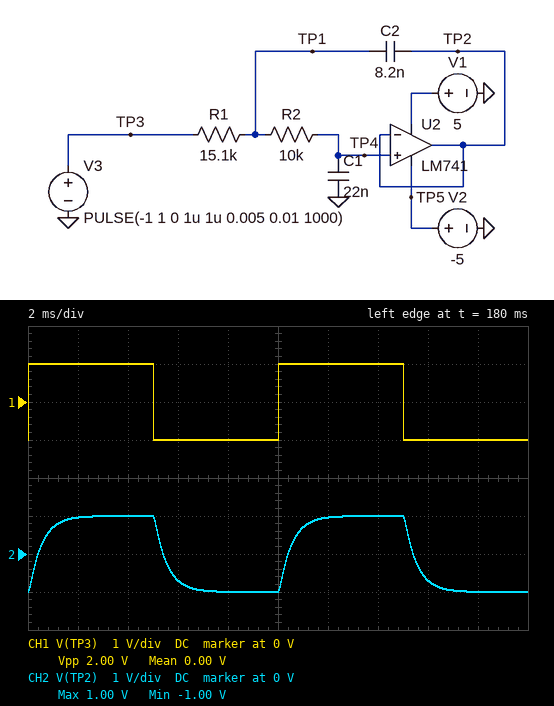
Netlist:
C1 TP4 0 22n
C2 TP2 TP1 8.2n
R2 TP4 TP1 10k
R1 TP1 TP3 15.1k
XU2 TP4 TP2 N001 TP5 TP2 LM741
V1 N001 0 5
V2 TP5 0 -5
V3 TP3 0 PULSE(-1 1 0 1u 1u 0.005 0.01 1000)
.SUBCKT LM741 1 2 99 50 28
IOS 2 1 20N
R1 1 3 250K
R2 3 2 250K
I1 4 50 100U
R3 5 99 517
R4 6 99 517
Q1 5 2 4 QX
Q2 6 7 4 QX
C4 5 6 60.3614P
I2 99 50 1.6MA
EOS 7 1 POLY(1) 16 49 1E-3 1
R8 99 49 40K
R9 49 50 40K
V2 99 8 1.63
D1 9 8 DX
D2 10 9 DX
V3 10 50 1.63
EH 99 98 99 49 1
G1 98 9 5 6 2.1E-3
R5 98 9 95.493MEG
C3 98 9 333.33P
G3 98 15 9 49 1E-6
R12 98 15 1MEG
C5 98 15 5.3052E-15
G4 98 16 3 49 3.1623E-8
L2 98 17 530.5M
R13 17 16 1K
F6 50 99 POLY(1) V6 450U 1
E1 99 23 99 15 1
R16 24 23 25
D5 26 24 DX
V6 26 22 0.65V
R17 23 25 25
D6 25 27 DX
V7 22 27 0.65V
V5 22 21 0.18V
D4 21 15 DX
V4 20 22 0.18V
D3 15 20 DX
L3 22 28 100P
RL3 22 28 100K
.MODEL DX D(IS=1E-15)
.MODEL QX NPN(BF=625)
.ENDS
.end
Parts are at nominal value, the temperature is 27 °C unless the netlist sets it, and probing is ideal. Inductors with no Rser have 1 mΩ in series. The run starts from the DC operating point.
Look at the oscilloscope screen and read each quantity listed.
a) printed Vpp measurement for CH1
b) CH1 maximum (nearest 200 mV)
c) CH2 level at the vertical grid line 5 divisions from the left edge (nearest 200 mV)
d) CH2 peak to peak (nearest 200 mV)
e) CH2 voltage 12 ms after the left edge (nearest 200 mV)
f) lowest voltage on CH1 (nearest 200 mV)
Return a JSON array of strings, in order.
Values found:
["2.00 V", "1.0 V", "-1.0 V", "2.0 V", "1.0 V", "-1.0 V"]
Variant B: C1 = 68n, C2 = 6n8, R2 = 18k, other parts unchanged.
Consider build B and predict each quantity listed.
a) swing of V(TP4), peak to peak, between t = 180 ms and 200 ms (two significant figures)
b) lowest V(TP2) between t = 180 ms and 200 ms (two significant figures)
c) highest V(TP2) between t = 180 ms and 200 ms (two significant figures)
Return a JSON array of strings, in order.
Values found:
["1.6 V", "-810 mV", "810 mV"]
